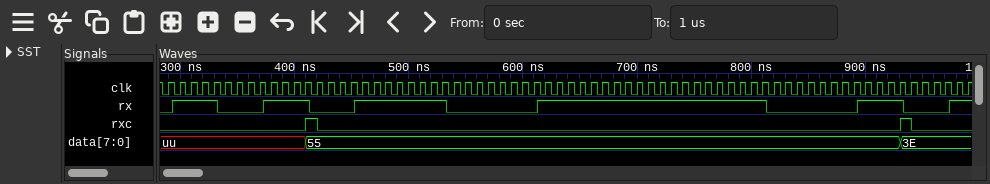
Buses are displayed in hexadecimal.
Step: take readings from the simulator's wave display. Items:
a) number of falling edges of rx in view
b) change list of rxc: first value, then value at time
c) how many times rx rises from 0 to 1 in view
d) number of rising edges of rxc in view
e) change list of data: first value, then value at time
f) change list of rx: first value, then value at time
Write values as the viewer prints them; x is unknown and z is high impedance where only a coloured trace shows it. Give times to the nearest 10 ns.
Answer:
5
0, 1 at 410 ns, 0 at 420 ns, 1 at 930 ns, 0 at 940 ns
6
2
uu, 55 at 410 ns, 3E at 930 ns
0, 1 at 290 ns, 0 at 330 ns, 1 at 370 ns, 0 at 410 ns, 1 at 450 ns, 0 at 530 ns, 1 at 610 ns, 0 at 810 ns, 1 at 890 ns, 0 at 930 ns, 1 at 970 ns
